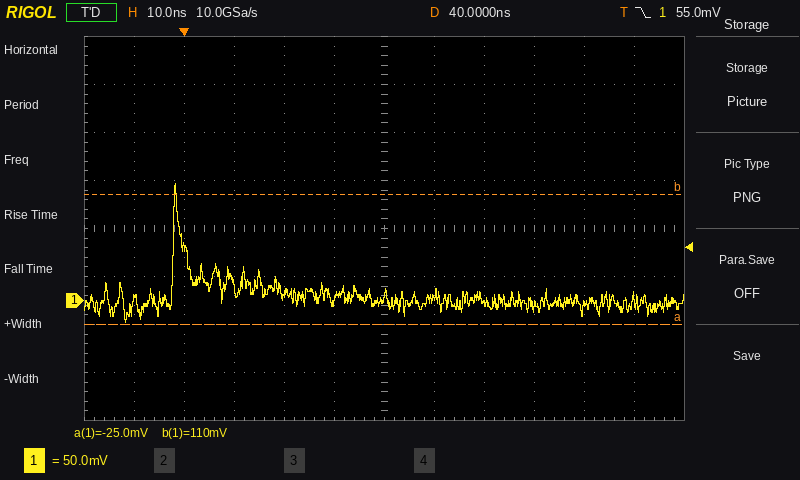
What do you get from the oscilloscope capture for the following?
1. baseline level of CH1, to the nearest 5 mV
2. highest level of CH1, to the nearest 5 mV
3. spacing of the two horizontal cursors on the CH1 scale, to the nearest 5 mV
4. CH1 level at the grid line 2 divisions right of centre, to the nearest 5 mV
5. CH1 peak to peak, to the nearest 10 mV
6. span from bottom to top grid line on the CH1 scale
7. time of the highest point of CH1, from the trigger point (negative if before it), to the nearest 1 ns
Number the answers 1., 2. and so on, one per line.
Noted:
1. 0 mV
2. 120 mV
3. 135 mV
4. 0 mV
5. 140 mV
6. 400 mV
7. -2 ns
